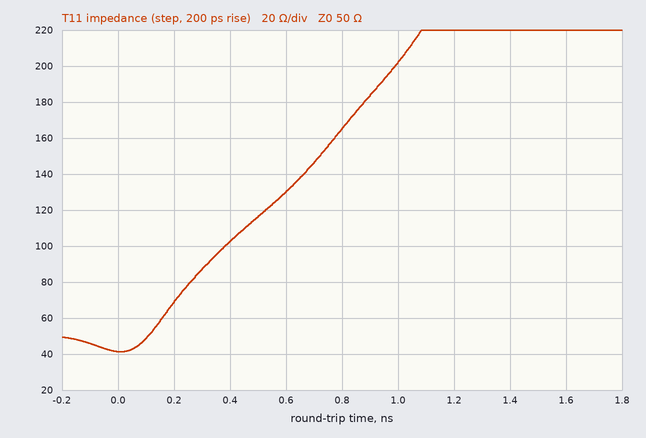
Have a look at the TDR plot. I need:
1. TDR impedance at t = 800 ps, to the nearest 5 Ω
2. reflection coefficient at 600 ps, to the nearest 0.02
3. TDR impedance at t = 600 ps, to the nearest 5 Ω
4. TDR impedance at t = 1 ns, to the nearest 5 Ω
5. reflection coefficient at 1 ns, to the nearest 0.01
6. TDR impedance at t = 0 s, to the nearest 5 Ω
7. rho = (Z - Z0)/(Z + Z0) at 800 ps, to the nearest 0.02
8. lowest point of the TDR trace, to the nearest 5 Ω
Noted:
165 Ω
+0.44
130 Ω
200 Ω
+0.60
40 Ω
+0.54
40 Ω
